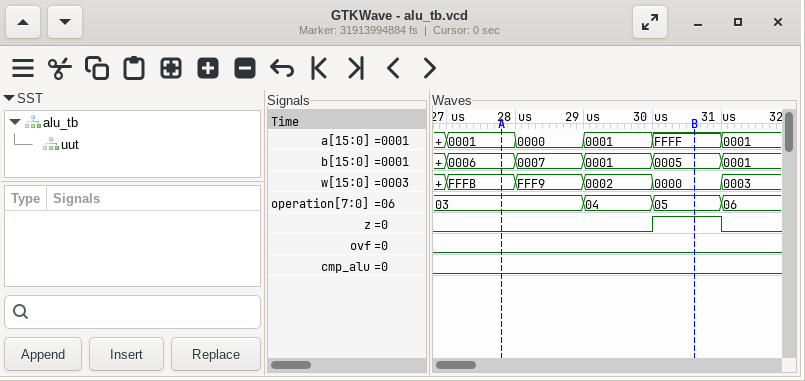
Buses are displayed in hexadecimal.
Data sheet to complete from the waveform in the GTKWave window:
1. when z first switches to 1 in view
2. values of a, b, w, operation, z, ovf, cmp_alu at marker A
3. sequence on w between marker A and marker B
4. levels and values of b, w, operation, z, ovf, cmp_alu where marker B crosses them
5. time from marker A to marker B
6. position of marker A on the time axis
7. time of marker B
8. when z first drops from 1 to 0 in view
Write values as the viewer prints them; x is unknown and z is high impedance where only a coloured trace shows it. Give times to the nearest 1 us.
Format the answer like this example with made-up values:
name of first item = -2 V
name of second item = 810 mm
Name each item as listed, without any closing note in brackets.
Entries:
when z first switches to 1 in view = 30 us
values of a, b, w, operation, z, ovf, cmp_alu at marker A = a=0001, b=0006, w=FFFB, operation=03, z=0, ovf=0, cmp_alu=0
sequence on w between marker A and marker B = FFFB, FFF9, 0002, 0000
levels and values of b, w, operation, z, ovf, cmp_alu where marker B crosses them = b=0005, w=0000, operation=05, z=1, ovf=0, cmp_alu=0
time from marker A to marker B = 3 us
position of marker A on the time axis = 28 us
time of marker B = 31 us
when z first drops from 1 to 0 in view = 31 us
